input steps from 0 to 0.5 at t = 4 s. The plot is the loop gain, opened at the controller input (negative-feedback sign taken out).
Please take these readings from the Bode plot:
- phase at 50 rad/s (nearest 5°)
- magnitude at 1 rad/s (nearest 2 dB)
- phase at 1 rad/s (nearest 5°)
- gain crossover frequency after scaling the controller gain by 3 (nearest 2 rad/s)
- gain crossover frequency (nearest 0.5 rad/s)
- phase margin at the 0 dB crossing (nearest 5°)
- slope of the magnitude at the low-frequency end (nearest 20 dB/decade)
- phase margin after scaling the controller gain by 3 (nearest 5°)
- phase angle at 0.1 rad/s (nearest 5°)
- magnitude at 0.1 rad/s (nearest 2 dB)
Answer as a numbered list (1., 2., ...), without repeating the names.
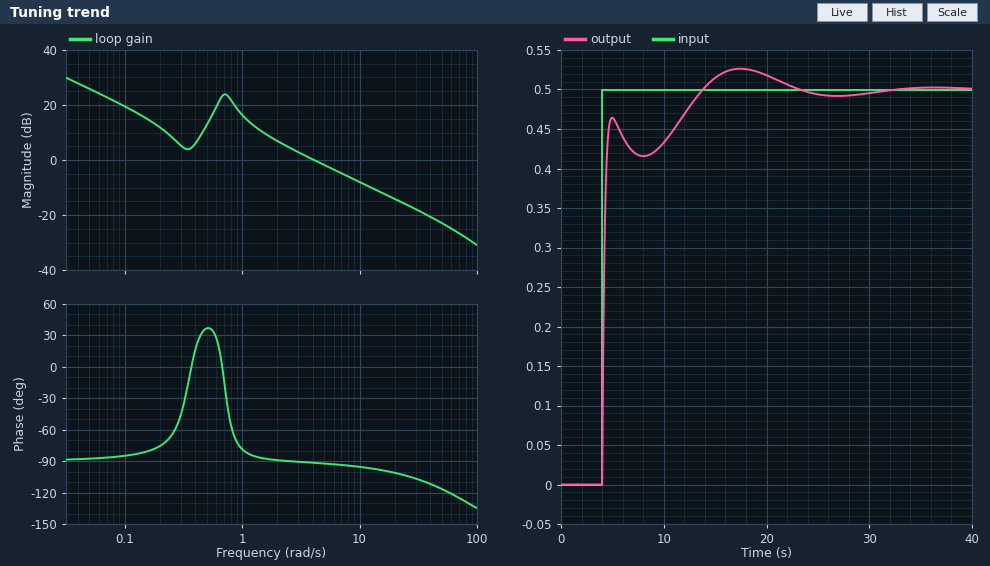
1. -115°
2. 16 dB
3. -80°
4. 12 rad/s
5. 4.0 rad/s
6. 90°
7. -20 dB/decade
8. 85°
9. -85°
10. 20 dB
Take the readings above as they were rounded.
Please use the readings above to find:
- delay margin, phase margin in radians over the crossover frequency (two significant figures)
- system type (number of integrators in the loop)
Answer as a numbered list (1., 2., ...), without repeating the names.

1. 0.39 s
2. 1
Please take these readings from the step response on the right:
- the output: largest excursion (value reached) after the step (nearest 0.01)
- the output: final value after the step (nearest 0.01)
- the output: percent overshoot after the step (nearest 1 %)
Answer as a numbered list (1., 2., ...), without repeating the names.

1. 0.53
2. 0.50
3. 5 %
